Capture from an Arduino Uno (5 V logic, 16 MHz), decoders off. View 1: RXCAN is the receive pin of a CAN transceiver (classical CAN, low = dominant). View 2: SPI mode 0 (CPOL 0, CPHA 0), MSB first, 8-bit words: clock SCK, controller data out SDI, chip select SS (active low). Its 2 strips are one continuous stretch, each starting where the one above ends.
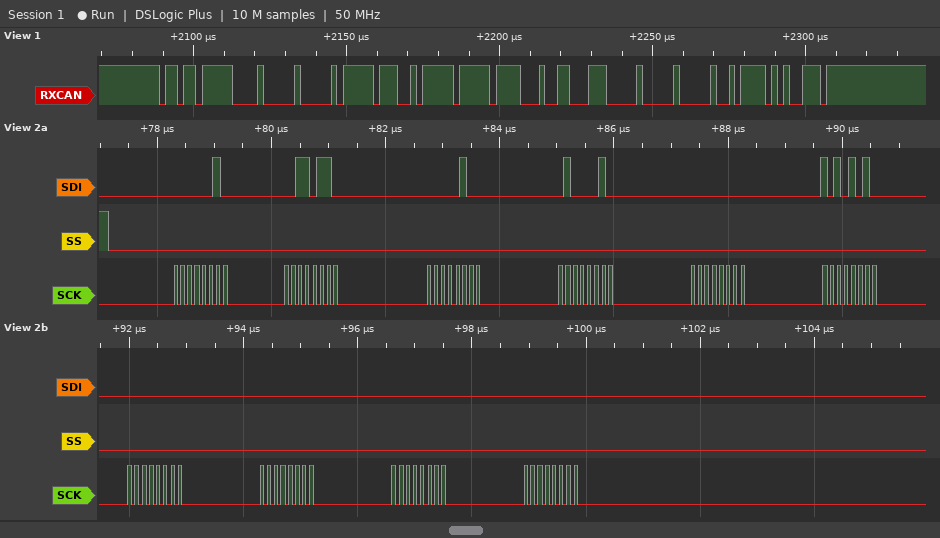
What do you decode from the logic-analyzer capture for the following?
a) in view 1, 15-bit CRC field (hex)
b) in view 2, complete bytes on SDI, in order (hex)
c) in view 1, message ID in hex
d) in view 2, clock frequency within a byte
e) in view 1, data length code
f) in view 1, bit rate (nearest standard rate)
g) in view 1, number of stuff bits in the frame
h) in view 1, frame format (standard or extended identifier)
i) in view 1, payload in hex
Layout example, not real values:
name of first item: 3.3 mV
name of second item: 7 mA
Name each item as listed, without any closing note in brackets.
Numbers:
in view 1, 15-bit CRC field: 0x2F53
in view 2, complete bytes on SDI, in order: 02 36 04 42 00 AA 00 00 00 00
in view 1, message ID in hex: 0x6DF
in view 2, clock frequency within a byte: 8 MHz
in view 1, data length code: 8
in view 1, bit rate: 500 kbit/s
in view 1, number of stuff bits in the frame: 9
in view 1, frame format: standard
in view 1, payload in hex: 00 FF 2F FF C4 C7 00 00
